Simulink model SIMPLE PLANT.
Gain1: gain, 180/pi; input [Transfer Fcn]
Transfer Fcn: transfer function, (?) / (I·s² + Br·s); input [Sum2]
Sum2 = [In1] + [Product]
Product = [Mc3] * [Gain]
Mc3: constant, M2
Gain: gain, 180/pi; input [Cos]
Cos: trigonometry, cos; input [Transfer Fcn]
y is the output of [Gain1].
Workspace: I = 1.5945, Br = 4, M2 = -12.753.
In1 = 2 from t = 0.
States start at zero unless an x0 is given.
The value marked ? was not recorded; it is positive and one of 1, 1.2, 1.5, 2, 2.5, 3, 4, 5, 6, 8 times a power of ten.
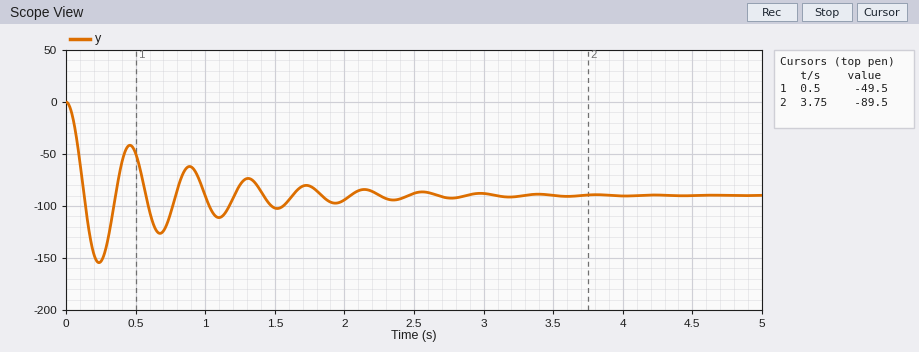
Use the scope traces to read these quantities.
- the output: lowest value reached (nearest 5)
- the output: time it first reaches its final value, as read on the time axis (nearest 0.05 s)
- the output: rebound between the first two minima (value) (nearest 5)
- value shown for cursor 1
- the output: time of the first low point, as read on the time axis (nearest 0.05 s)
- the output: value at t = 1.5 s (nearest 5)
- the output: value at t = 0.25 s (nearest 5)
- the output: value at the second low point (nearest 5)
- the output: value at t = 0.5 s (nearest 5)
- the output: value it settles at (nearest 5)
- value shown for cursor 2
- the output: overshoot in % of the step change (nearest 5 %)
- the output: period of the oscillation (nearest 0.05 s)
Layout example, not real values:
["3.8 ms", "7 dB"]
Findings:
["-155", "0.15 s", "-40", "-49.5", "0.25 s", "-100", "-155", "-125", "-50", "-90", "-89.5", "70 %", "0.45 s"]
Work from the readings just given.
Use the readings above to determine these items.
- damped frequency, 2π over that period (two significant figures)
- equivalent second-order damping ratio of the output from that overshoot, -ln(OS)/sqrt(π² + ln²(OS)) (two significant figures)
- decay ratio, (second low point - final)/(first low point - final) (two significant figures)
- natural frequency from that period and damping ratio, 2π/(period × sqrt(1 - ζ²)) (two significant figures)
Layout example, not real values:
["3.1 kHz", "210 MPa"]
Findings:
["14 rad/s", "0.11", "0.54", "14 rad/s"]
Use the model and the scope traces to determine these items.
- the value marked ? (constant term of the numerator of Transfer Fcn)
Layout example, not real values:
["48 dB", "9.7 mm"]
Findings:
["0.5"]
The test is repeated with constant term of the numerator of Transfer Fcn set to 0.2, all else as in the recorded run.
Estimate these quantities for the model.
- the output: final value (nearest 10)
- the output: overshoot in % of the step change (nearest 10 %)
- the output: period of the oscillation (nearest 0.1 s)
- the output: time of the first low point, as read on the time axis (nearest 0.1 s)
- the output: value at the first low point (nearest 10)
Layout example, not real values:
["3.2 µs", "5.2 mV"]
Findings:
["-90", "60 %", "0.7 s", "0.4 s", "-140"]
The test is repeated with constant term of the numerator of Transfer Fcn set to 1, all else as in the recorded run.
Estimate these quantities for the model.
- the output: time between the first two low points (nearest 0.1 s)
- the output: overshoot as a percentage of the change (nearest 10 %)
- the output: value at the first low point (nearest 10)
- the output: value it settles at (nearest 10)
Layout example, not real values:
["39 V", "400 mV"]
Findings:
["0.3 s", "80 %", "-160", "-90"]
